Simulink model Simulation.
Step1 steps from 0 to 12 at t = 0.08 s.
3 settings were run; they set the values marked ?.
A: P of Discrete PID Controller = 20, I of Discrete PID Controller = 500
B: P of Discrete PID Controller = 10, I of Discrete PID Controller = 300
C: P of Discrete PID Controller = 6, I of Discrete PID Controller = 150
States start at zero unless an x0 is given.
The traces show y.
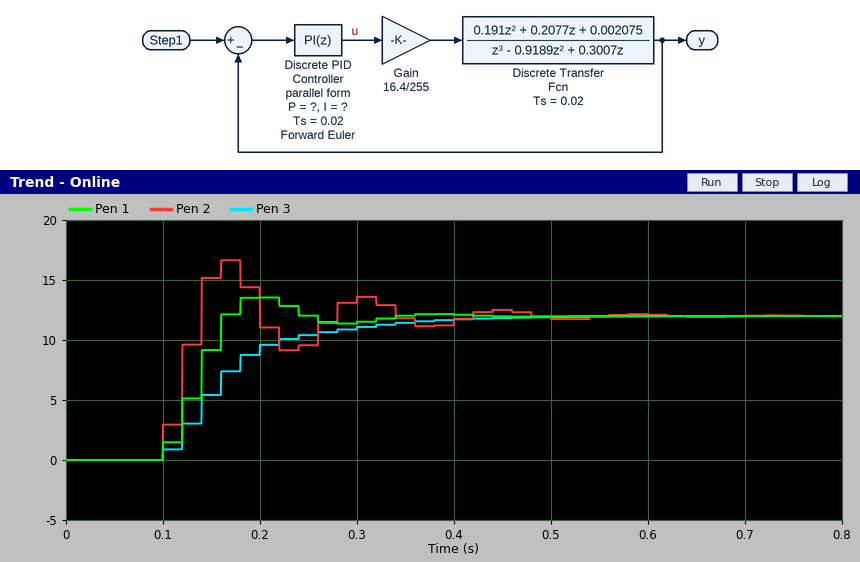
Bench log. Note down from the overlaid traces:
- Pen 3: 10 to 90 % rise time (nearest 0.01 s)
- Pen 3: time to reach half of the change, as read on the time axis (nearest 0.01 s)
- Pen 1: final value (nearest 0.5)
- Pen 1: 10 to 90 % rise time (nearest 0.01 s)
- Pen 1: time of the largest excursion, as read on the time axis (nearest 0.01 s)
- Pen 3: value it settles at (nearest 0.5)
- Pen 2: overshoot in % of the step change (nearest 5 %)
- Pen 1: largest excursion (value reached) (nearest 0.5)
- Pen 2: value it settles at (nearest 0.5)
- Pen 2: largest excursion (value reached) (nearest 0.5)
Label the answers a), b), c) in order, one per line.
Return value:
a) 0.16 s
b) 0.16 s
c) 12.0
d) 0.06 s
e) 0.20 s
f) 12.0
g) 40 %
h) 13.5
i) 12.0
j) 16.5
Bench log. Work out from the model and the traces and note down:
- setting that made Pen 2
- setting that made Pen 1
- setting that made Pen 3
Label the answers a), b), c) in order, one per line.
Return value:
a) A
b) B
c) C
